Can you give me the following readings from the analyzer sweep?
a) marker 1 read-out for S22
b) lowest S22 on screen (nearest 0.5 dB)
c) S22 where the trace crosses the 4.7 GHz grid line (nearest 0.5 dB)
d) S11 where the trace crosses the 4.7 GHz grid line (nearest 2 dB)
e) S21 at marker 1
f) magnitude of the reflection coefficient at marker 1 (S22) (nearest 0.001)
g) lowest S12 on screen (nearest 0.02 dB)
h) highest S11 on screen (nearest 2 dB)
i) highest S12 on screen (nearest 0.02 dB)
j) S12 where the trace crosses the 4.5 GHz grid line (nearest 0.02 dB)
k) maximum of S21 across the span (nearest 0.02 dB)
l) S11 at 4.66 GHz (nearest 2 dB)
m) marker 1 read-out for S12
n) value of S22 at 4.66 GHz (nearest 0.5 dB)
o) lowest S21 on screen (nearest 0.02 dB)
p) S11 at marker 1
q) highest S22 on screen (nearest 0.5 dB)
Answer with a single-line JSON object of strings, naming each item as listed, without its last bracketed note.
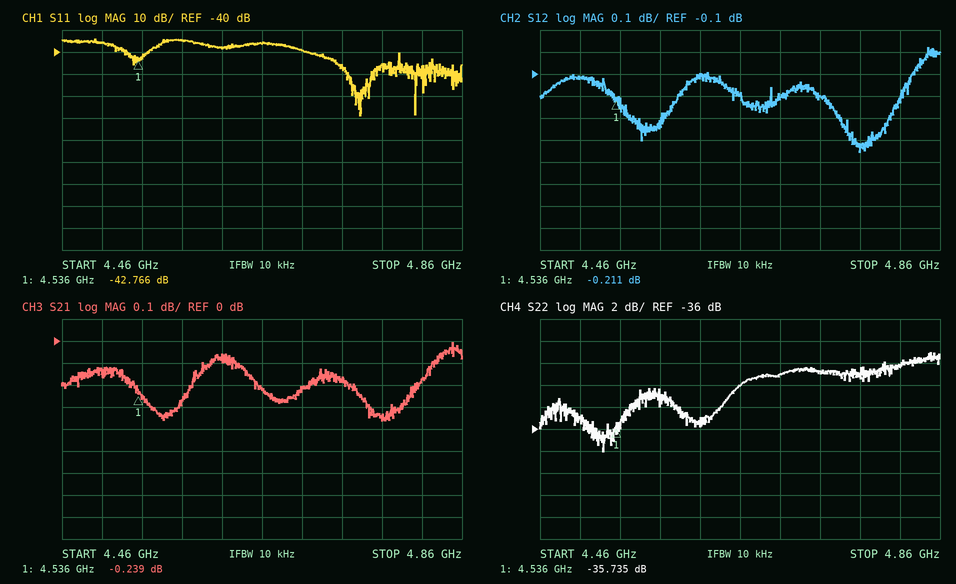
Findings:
{"marker 1 read-out for S22": "-35.735 dB", "lowest S22 on screen": "-38.0 dB", "S22 where the trace crosses the 4.7 GHz grid line": "-31.0 dB", "S11 where the trace crosses the 4.7 GHz grid line": "-40 dB", "S21 at marker 1": "-0.239 dB", "magnitude of the reflection coefficient at marker 1 (S22)": "0.016", "lowest S12 on screen": "-0.46 dB", "highest S11 on screen": "-34 dB", "highest S12 on screen": "0.02 dB", "S12 where the trace crosses the 4.5 GHz grid line": "-0.12 dB", "maximum of S21 across the span": "0.00 dB", "S11 at 4.66 GHz": "-36 dB", "marker 1 read-out for S12": "-0.211 dB", "value of S22 at 4.66 GHz": "-32.0 dB", "lowest S21 on screen": "-0.36 dB", "S11 at marker 1": "-42.766 dB", "highest S22 on screen": "-29.0 dB"}
